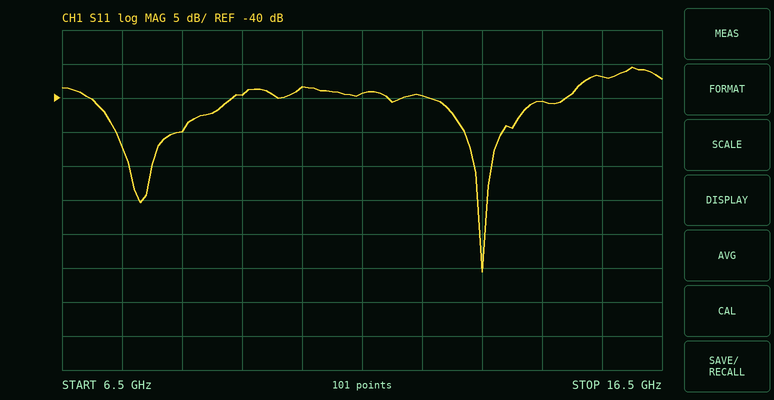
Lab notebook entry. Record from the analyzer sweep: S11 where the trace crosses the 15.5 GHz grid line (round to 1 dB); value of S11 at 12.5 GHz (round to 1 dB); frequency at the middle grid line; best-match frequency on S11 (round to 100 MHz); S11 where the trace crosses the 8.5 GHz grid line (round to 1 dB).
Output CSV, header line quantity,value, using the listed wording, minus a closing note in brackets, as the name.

quantity,value
S11 where the trace crosses the 15.5 GHz grid line,-37 dB
value of S11 at 12.5 GHz,-40 dB
frequency at the middle grid line,11.5 GHz
best-match frequency on S11,13.5 GHz
S11 where the trace crosses the 8.5 GHz grid line,-45 dB
